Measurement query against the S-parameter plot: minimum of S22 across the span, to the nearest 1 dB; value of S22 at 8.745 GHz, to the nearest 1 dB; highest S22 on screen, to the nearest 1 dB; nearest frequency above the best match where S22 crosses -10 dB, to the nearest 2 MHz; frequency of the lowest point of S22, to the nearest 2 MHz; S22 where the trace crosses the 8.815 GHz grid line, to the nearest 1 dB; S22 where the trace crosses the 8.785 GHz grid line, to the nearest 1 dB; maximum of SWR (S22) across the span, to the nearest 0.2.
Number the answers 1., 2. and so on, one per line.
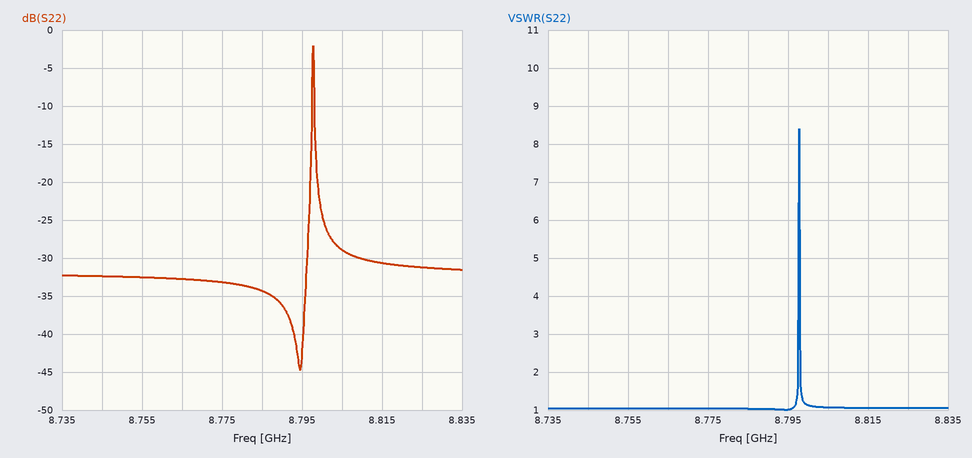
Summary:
1. -45 dB
2. -32 dB
3. -2 dB
4. 8.798 GHz
5. 8.794 GHz
6. -31 dB
7. -34 dB
8. 8.4
